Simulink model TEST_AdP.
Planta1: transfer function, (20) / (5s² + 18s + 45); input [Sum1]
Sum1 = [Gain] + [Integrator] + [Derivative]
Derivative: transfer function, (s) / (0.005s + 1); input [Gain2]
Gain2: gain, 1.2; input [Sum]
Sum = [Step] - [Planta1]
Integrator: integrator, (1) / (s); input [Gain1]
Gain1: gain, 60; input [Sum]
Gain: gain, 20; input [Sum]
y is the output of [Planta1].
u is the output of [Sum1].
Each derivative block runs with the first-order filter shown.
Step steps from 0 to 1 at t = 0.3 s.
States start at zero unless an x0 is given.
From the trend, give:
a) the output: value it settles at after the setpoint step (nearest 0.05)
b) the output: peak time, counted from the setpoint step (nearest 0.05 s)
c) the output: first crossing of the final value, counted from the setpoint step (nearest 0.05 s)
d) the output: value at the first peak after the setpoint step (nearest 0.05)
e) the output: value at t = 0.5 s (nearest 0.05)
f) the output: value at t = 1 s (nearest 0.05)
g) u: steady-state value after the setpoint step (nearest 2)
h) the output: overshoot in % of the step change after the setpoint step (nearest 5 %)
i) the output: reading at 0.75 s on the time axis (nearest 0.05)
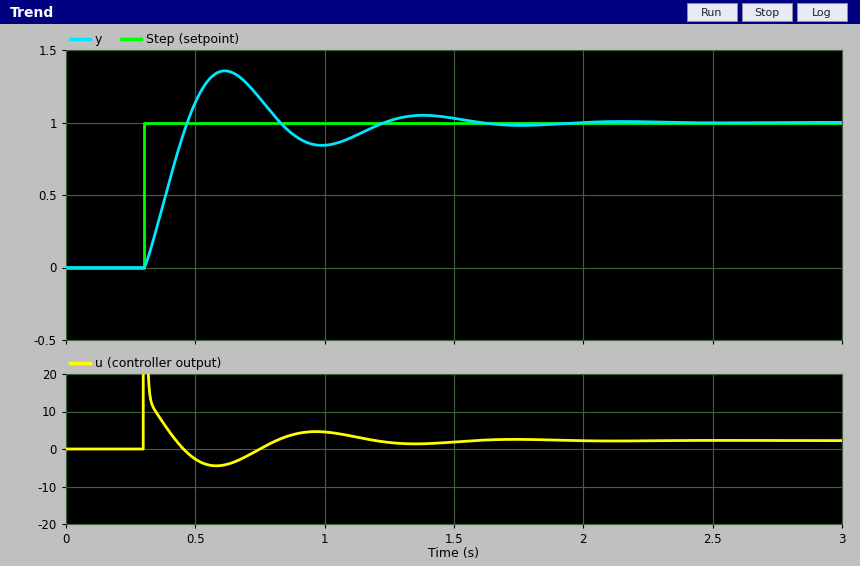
1.00
0.30 s
0.15 s
1.35
1.15
0.85
2
35 %
1.15
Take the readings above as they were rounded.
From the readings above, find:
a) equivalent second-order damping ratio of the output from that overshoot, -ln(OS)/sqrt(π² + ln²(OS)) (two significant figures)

0.32
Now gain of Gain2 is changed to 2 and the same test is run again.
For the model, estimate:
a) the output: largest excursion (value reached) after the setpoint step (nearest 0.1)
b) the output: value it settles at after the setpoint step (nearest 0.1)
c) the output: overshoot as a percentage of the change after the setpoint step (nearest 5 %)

1.2
1.0
20 %
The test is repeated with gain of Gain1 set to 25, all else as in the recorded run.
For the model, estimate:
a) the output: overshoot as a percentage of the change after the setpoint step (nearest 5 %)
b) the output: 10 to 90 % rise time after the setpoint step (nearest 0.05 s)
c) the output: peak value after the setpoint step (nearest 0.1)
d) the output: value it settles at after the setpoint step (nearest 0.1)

25 %
0.15 s
1.2
1.0
